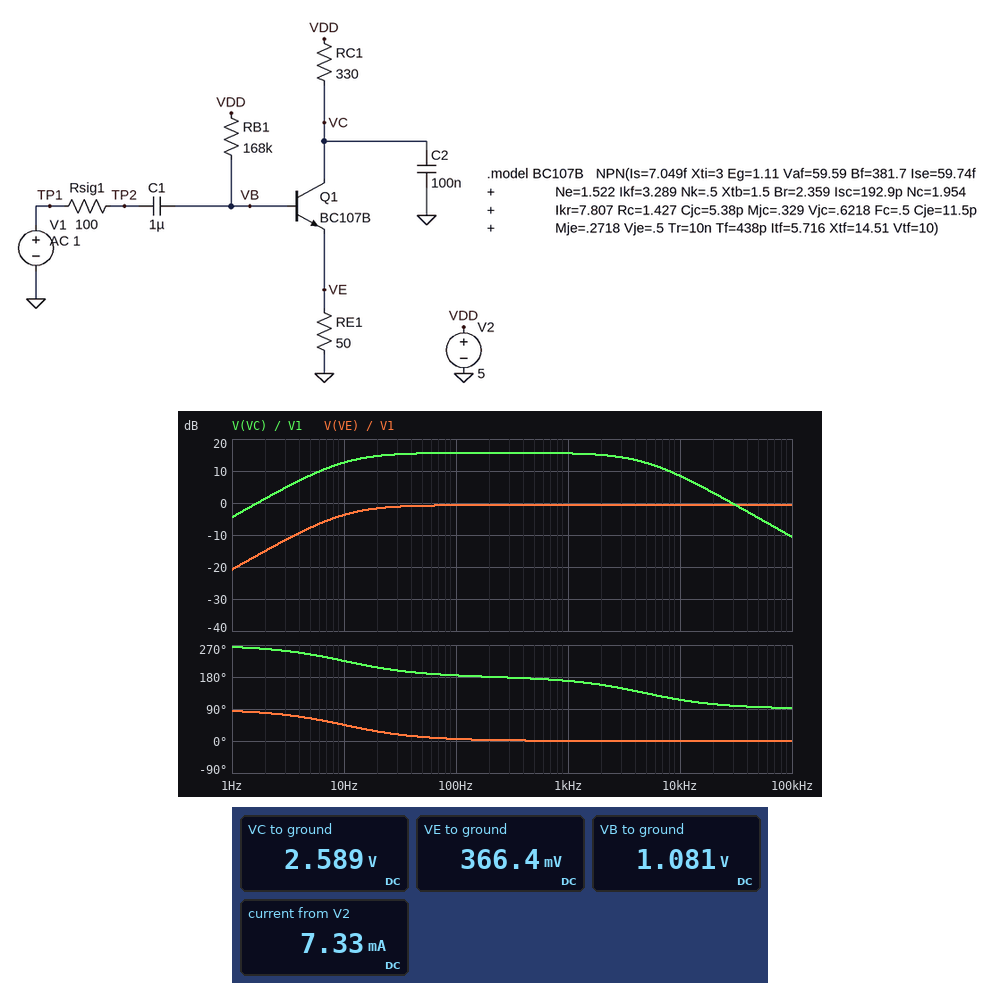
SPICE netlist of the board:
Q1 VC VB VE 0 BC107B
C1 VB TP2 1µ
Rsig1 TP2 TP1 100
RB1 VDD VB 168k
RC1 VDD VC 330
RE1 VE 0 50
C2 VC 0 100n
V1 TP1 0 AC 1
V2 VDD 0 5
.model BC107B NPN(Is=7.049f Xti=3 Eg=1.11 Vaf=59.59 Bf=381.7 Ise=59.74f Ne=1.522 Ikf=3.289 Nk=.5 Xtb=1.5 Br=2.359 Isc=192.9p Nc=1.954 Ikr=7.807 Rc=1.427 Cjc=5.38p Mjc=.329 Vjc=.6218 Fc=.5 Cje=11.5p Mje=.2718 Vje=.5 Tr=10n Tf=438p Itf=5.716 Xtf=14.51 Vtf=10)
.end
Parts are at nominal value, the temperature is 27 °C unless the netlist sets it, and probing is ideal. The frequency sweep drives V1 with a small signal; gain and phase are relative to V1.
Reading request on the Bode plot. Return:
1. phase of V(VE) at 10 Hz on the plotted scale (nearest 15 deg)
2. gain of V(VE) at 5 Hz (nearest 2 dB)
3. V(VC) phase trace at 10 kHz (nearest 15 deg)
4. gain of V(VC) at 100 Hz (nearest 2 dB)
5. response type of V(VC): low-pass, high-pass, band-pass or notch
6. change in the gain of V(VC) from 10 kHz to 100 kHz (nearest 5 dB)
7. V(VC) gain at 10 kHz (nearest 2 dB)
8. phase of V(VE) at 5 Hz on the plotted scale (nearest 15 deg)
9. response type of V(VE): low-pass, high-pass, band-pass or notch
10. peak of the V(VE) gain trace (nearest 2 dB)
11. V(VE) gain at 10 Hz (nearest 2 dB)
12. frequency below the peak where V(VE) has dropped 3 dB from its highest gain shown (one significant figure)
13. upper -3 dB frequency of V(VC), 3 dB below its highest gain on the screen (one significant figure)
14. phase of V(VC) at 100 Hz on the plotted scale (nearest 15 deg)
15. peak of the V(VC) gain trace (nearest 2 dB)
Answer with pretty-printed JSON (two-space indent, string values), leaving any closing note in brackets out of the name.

{
  "phase of V(VE) at 10 Hz on the plotted scale": "45 deg",
  "gain of V(VE) at 5 Hz": "-8 dB",
  "V(VC) phase trace at 10 kHz": "120 deg",
  "gain of V(VC) at 100 Hz": "16 dB",
  "response type of V(VC): low-pass, high-pass, band-pass or notch": "band-pass",
  "change in the gain of V(VC) from 10 kHz to 100 kHz": "-20 dB",
  "V(VC) gain at 10 kHz": "8 dB",
  "phase of V(VE) at 5 Hz on the plotted scale": "60 deg",
  "response type of V(VE): low-pass, high-pass, band-pass or notch": "high-pass",
  "peak of the V(VE) gain trace": "0 dB",
  "V(VE) gain at 10 Hz": "-4 dB",
  "frequency below the peak where V(VE) has dropped 3 dB from its highest gain shown": "10 Hz",
  "upper -3 dB frequency of V(VC), 3 dB below its highest gain on the screen": "5 kHz",
  "phase of V(VC) at 100 Hz on the plotted scale": "180 deg",
  "peak of the V(VC) gain trace": "16 dB"
}
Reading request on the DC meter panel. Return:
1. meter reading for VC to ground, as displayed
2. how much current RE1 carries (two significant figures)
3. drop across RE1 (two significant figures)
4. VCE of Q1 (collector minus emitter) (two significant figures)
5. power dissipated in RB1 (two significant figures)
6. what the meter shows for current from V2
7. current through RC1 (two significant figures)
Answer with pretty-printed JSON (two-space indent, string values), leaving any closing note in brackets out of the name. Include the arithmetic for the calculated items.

{
  "meter reading for VC to ground, as displayed": "2.589 V",
  "how much current RE1 carries": "(366.4 mV) / 50 Ω = 7.3 mA",
  "drop across RE1": "366.4 mV = 370 mV",
  "VCE of Q1 (collector minus emitter)": "2.589 V - 366.4 mV = 2.2 V",
  "power dissipated in RB1": "(5 V - 1.081 V)^2 / 168 kΩ = 91 µW",
  "what the meter shows for current from V2": "7.33 mA",
  "current through RC1": "(5 V - 2.589 V) / 330 Ω = 7.3 mA"
}
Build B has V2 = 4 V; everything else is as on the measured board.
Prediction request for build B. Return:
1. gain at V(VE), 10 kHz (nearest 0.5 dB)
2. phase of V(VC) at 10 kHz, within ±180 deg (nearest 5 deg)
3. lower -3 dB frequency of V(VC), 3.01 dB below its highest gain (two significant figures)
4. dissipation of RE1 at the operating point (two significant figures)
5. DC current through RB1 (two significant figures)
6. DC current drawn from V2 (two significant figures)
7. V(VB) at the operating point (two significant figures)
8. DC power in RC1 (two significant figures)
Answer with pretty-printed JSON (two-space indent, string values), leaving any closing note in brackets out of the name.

{
  "gain at V(VE), 10 kHz": "-1.0 dB",
  "phase of V(VC) at 10 kHz, within ±180 deg": "115 deg",
  "lower -3 dB frequency of V(VC), 3.01 dB below its highest gain": "9.9 Hz",
  "dissipation of RE1 at the operating point": "1.5 mW",
  "DC current through RB1": "18 µA",
  "DC current drawn from V2": "5.5 mA",
  "V(VB) at the operating point": "980 mV",
  "DC power in RC1": "9.9 mW"
}
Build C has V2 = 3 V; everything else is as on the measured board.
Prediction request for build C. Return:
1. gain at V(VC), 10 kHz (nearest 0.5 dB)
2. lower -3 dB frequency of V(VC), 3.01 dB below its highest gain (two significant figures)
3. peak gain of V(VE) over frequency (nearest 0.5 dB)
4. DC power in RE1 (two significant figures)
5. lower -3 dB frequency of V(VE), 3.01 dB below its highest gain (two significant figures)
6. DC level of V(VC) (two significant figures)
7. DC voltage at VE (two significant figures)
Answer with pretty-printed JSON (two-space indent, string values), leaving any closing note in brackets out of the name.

{
  "gain at V(VC), 10 kHz": "8.0 dB",
  "lower -3 dB frequency of V(VC), 3.01 dB below its highest gain": "9.7 Hz",
  "peak gain of V(VE) over frequency": "-1.0 dB",
  "DC power in RE1": "700 µW",
  "lower -3 dB frequency of V(VE), 3.01 dB below its highest gain": "9.8 Hz",
  "DC level of V(VC)": "1.8 V",
  "DC voltage at VE": "190 mV"
}
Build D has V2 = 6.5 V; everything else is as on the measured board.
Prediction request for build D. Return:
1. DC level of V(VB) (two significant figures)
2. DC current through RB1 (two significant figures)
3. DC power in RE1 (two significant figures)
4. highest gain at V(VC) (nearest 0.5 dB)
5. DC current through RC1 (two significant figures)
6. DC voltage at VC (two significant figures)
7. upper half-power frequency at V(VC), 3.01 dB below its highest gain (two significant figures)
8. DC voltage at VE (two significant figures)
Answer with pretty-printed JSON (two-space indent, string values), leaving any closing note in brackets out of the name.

{
  "DC level of V(VB)": "1.2 V",
  "DC current through RB1": "31 µA",
  "DC power in RE1": "5.1 mW",
  "highest gain at V(VC)": "16.0 dB",
  "DC current through RC1": "10 mA",
  "DC voltage at VC": "3.2 V",
  "upper half-power frequency at V(VC), 3.01 dB below its highest gain": "4.9 kHz",
  "DC voltage at VE": "510 mV"
}
